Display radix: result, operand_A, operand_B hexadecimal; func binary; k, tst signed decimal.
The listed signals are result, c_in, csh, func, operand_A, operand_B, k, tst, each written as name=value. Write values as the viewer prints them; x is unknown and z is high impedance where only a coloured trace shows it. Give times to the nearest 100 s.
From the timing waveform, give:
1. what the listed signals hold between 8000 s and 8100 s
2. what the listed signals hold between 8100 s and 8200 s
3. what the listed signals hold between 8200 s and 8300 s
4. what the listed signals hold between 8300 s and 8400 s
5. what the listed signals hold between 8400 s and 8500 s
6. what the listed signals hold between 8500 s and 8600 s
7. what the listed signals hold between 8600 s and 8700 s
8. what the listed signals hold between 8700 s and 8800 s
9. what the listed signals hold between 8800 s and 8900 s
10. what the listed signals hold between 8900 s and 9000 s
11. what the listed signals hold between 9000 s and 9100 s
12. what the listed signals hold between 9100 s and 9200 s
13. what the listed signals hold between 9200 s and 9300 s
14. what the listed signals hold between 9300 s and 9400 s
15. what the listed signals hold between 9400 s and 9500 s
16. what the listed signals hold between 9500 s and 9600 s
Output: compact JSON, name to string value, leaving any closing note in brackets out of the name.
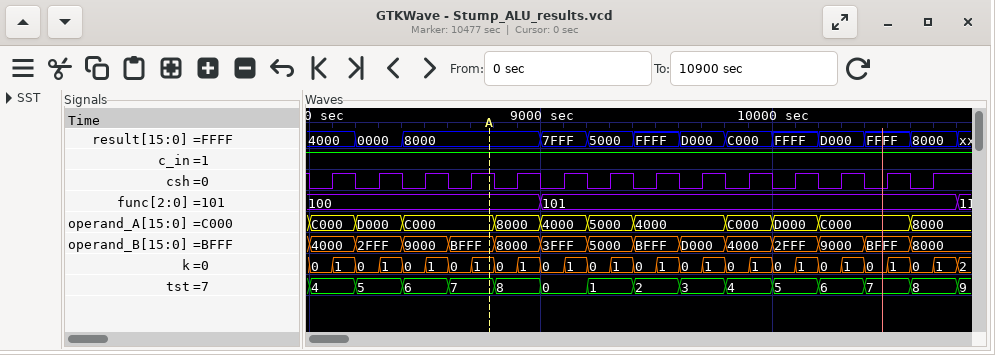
{"what the listed signals hold between 8000 s and 8100 s": "result=4000, c_in=1, csh=0, func=100, operand_A=C000, operand_B=4000, k=0, tst=4", "what the listed signals hold between 8100 s and 8200 s": "result=4000, c_in=1, csh=1, func=100, operand_A=C000, operand_B=4000, k=1, tst=4", "what the listed signals hold between 8200 s and 8300 s": "result=0000, c_in=1, csh=0, func=100, operand_A=D000, operand_B=2FFF, k=0, tst=5", "what the listed signals hold between 8300 s and 8400 s": "result=0000, c_in=1, csh=1, func=100, operand_A=D000, operand_B=2FFF, k=1, tst=5", "what the listed signals hold between 8400 s and 8500 s": "result=8000, c_in=1, csh=0, func=100, operand_A=C000, operand_B=9000, k=0, tst=6", "what the listed signals hold between 8500 s and 8600 s": "result=8000, c_in=1, csh=1, func=100, operand_A=C000, operand_B=9000, k=1, tst=6", "what the listed signals hold between 8600 s and 8700 s": "result=8000, c_in=1, csh=0, func=100, operand_A=C000, operand_B=BFFF, k=0, tst=7", "what the listed signals hold between 8700 s and 8800 s": "result=8000, c_in=1, csh=1, func=100, operand_A=C000, operand_B=BFFF, k=1, tst=7", "what the listed signals hold between 8800 s and 8900 s": "result=8000, c_in=1, csh=0, func=100, operand_A=8000, operand_B=8000, k=0, tst=8", "what the listed signals hold between 8900 s and 9000 s": "result=8000, c_in=1, csh=1, func=100, operand_A=8000, operand_B=8000, k=1, tst=8", "what the listed signals hold between 9000 s and 9100 s": "result=7FFF, c_in=1, csh=0, func=101, operand_A=4000, operand_B=3FFF, k=0, tst=0", "what the listed signals hold between 9100 s and 9200 s": "result=7FFF, c_in=1, csh=1, func=101, operand_A=4000, operand_B=3FFF, k=1, tst=0", "what the listed signals hold between 9200 s and 9300 s": "result=5000, c_in=1, csh=0, func=101, operand_A=5000, operand_B=5000, k=0, tst=1", "what the listed signals hold between 9300 s and 9400 s": "result=5000, c_in=1, csh=1, func=101, operand_A=5000, operand_B=5000, k=1, tst=1", "what the listed signals hold between 9400 s and 9500 s": "result=FFFF, c_in=1, csh=0, func=101, operand_A=4000, operand_B=BFFF, k=0, tst=2", "what the listed signals hold between 9500 s and 9600 s": "result=FFFF, c_in=1, csh=1, func=101, operand_A=4000, operand_B=BFFF, k=1, tst=2"}
